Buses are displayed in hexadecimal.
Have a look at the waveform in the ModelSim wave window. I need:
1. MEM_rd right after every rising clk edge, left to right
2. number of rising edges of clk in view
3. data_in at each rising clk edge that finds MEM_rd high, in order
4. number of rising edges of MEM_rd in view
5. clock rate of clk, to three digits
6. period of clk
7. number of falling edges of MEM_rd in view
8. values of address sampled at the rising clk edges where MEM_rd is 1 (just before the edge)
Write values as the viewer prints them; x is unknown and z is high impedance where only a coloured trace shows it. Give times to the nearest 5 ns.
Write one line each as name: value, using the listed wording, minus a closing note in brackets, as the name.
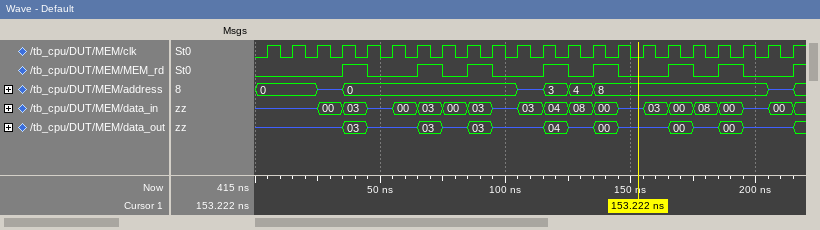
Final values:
MEM_rd right after every rising clk edge, left to right: 0 0 0 1 0 0 1 0 1 0 0 1 0 1 0 0 1 0 1 0 0 1
number of rising edges of clk in view: 22
data_in at each rising clk edge that finds MEM_rd high, in order: 03, 03, 03, 04, 00, 00, 00
number of rising edges of MEM_rd in view: 8
clock rate of clk, to three digits: 100 MHz
period of clk: 10 ns
number of falling edges of MEM_rd in view: 7
values of address sampled at the rising clk edges where MEM_rd is 1: 0, 0, 0, 3, 8, 8, 8
